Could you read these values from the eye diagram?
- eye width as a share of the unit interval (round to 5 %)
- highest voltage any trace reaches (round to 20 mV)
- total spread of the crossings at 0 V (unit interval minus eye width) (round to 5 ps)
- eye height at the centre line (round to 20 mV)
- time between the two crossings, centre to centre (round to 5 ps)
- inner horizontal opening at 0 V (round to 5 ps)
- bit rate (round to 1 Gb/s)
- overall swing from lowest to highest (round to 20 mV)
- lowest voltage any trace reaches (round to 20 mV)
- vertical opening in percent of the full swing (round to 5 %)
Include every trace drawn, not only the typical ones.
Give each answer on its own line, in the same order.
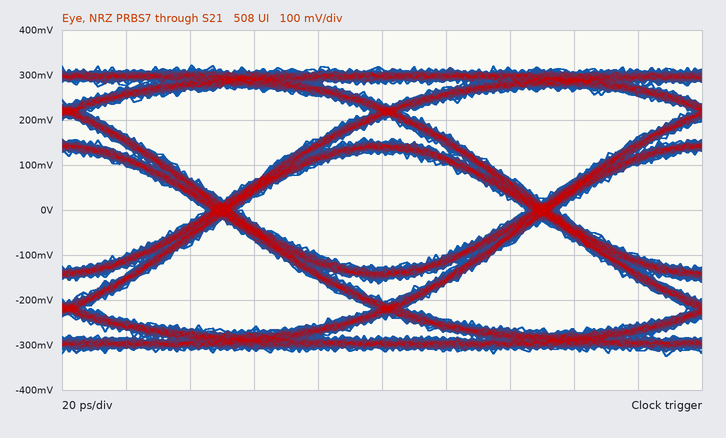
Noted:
90 %
320 mV
10 ps
260 mV
100 ps
90 ps
10 Gb/s
640 mV
-320 mV
40 %
